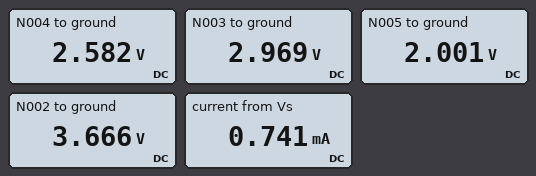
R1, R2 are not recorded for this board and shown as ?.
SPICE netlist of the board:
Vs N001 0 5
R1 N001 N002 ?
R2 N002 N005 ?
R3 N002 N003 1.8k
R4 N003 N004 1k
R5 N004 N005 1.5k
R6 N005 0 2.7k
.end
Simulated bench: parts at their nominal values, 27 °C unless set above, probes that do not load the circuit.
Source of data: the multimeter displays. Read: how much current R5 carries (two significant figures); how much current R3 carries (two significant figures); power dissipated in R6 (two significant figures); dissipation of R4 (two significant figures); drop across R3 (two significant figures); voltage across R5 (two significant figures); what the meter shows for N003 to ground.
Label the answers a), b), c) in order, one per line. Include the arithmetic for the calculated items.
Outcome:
a) (2.582 V - 2.001 V) / 1.5 kΩ = 390 µA
b) (3.666 V - 2.969 V) / 1.8 kΩ = 390 µA
c) (2.001 V)^2 / 2.7 kΩ = 1.5 mW
d) (2.969 V - 2.582 V)^2 / 1 kΩ = 150 µW
e) 3.666 V - 2.969 V = 700 mV
f) 2.582 V - 2.001 V = 580 mV
g) 2.969 V
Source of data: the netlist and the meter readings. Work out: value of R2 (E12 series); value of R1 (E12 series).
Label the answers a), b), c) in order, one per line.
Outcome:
a) 4.7 kΩ
b) 1.8 kΩ
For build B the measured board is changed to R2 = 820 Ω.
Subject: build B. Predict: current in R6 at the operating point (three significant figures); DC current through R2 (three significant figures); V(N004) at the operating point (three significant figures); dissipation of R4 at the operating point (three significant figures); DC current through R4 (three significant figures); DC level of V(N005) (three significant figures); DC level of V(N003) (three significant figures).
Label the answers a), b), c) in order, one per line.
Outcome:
a) 964 µA
b) 809 µA
c) 2.83 V
d) 23.8 µW
e) 154 µA
f) 2.60 V
g) 2.99 V
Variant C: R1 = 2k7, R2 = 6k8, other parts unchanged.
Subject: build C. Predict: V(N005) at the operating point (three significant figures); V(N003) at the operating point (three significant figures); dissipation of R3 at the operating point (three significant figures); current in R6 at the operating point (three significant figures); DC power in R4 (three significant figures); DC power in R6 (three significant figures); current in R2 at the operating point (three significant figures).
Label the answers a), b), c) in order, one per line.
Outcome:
a) 1.68 V
b) 2.63 V
c) 262 µW
d) 622 µA
e) 145 µW
f) 1.05 mW
g) 241 µA
